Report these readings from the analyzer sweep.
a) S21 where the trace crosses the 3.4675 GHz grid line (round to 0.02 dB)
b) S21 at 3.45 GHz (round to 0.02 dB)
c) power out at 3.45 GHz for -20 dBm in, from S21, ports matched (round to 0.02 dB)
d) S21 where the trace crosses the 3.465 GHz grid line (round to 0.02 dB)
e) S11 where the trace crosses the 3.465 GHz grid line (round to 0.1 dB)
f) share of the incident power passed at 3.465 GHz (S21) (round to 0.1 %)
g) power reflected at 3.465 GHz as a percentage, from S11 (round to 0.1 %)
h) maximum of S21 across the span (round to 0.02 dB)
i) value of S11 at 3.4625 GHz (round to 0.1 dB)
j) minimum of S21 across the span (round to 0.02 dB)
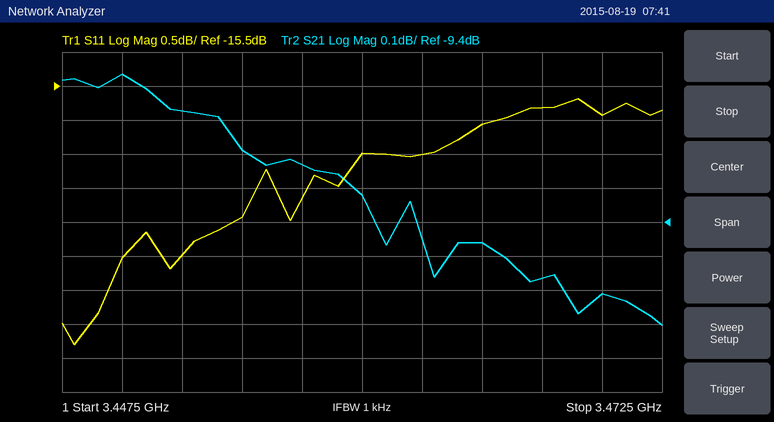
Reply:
-9.56 dB
-8.96 dB
-28.96 dBm
-9.46 dB
-16.1 dB
11.3 %
2.5 %
-8.96 dB
-16.5 dB
-9.70 dB
